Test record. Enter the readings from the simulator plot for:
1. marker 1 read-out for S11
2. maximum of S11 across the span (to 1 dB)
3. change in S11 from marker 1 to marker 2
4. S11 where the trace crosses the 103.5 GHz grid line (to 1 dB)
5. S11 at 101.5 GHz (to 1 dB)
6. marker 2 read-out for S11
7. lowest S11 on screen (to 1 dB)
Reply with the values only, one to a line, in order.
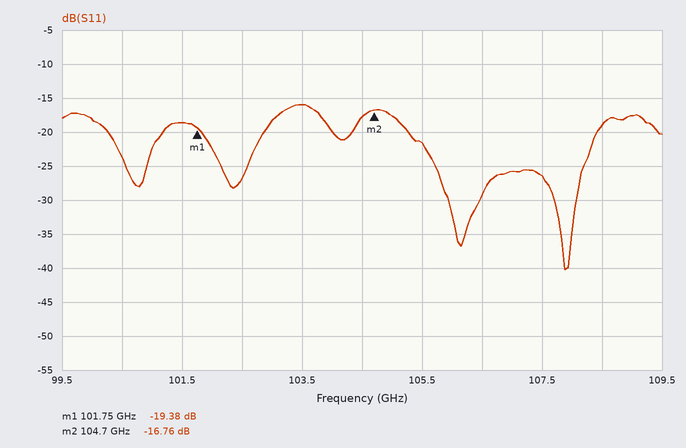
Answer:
-19.38 dB
-16 dB
2.62 dB
-16 dB
-19 dB
-16.76 dB
-40 dB
